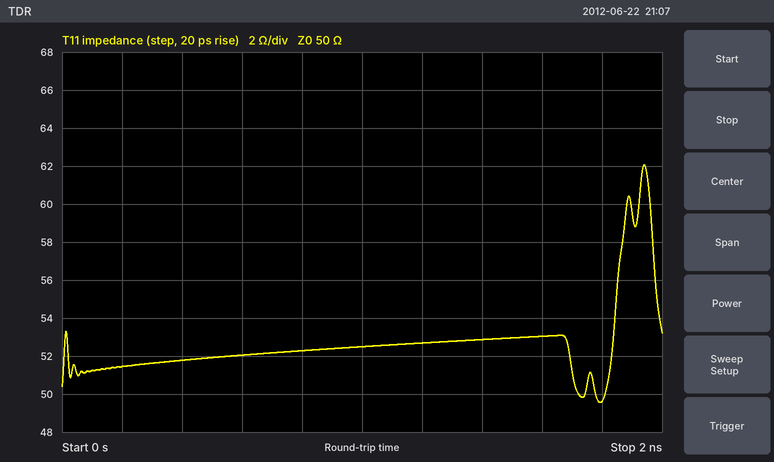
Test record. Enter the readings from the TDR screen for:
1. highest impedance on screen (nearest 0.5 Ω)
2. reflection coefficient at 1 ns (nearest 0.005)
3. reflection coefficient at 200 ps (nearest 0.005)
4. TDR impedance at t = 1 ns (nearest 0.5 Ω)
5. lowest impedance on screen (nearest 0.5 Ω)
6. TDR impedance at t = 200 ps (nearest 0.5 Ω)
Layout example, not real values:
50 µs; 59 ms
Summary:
62.0 Ω; +0.025; +0.015; 52.5 Ω; 49.5 Ω; 51.5 Ω
